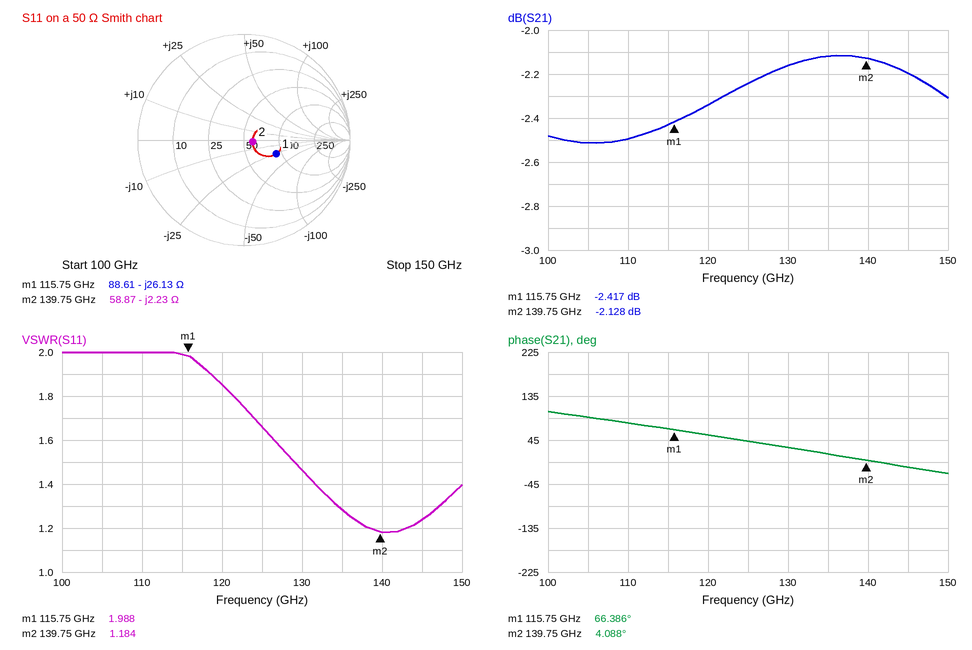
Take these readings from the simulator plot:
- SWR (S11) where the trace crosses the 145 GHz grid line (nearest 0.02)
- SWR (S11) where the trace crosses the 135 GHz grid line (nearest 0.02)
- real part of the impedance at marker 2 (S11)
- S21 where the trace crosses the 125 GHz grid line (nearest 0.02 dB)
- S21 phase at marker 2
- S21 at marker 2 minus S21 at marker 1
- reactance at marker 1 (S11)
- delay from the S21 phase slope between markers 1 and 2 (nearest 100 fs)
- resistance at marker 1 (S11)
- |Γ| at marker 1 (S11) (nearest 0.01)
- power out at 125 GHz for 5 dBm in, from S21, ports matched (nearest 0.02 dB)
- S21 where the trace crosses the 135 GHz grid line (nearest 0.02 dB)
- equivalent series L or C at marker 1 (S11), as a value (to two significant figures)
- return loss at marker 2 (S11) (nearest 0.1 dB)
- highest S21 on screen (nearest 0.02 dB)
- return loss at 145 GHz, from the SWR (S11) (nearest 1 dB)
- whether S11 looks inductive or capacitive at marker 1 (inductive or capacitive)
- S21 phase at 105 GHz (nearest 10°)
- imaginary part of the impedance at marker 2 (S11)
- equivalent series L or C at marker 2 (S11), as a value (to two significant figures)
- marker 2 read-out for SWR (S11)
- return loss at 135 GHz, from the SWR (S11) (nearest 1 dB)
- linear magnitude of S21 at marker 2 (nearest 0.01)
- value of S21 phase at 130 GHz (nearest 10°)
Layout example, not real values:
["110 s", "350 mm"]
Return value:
["1.24", "1.28", "58.87 Ω", "-2.24 dB", "4.088°", "0.289 dB", "-26.13 Ω", "7.2 ps", "88.61 Ω", "0.33", "2.76 dBm", "-2.12 dB", "53 fF", "21.5 dB", "-2.12 dB", "19 dB", "capacitive", "90°", "-2.23 Ω", "510 fF", "1.184", "18 dB", "0.78", "30°"]
